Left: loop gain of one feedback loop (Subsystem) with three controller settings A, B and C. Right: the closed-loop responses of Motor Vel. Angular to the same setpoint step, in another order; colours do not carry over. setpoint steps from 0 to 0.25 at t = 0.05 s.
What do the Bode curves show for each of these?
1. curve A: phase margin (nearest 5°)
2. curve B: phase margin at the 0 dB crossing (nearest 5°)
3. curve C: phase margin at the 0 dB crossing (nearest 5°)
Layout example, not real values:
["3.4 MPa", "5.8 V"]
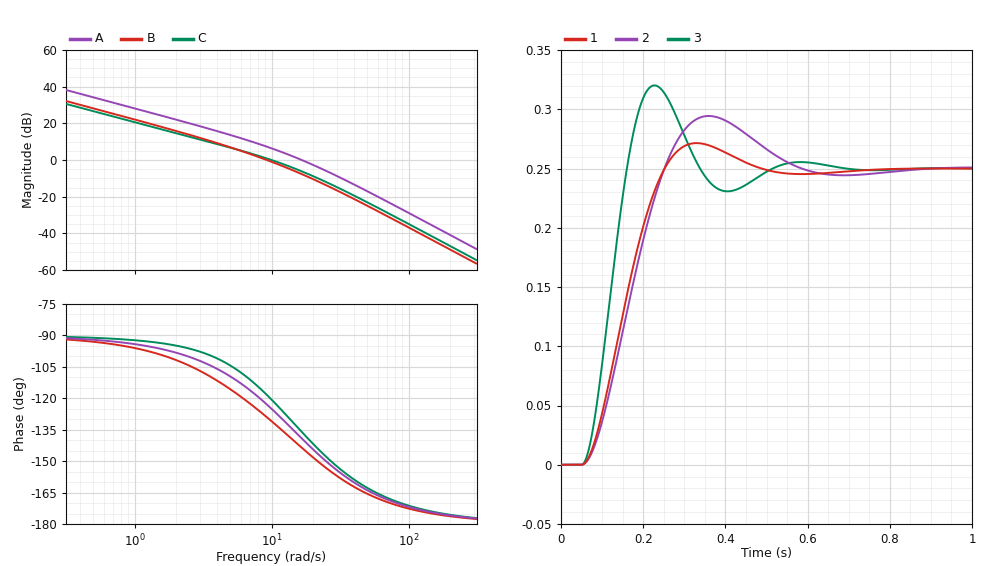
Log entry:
["40°", "50°", "60°"]
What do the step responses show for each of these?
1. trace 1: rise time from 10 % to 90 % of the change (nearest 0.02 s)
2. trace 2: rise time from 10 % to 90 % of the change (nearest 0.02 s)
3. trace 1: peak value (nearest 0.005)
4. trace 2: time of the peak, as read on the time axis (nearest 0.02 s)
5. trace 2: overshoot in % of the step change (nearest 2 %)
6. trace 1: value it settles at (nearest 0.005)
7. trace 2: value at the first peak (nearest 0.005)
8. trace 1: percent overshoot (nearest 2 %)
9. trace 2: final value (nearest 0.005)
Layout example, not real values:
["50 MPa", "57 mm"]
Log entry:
["0.14 s", "0.14 s", "0.270", "0.36 s", "18 %", "0.250", "0.295", "8 %", "0.250"]
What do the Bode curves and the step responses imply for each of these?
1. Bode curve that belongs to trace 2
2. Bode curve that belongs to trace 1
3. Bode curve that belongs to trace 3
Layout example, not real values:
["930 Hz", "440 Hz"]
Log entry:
["B", "C", "A"]
